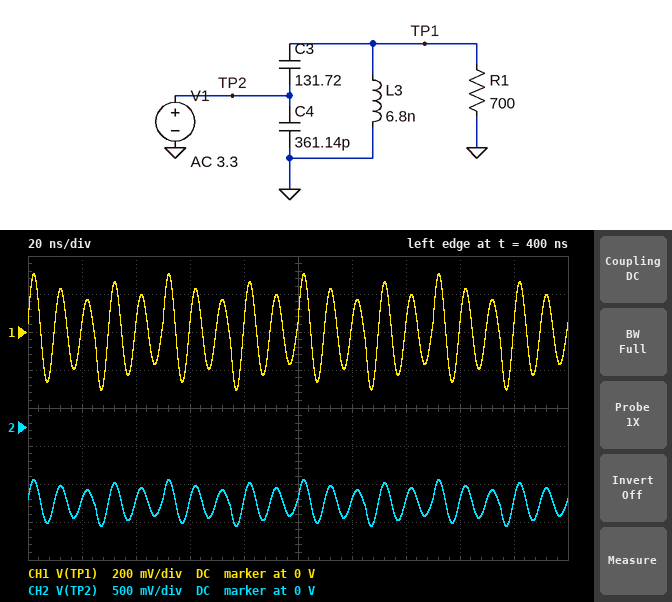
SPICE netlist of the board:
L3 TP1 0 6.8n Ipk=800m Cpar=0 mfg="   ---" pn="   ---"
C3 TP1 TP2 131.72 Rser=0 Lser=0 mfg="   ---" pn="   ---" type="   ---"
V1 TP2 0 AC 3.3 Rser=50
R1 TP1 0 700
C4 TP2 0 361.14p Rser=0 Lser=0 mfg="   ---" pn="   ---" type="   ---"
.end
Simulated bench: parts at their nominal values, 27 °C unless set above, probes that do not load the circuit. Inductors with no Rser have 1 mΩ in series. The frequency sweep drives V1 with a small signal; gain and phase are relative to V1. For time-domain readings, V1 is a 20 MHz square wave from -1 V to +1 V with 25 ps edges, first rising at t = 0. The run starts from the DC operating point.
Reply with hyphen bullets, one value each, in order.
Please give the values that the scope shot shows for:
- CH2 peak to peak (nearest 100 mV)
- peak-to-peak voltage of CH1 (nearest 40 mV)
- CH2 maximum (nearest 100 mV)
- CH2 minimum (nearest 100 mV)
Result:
- 600 mV
- 600 mV
- -700 mV
- -1.3 V
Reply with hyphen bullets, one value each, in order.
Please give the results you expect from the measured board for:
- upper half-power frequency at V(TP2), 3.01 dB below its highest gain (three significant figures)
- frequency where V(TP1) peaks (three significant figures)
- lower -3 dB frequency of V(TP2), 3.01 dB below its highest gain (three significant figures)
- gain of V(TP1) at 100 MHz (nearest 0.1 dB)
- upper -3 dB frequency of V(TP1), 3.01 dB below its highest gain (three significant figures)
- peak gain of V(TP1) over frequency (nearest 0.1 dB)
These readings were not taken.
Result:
- 106 MHz
- 102 MHz
- 96.9 MHz
- -1.1 dB
- 106 MHz
- -0.6 dB
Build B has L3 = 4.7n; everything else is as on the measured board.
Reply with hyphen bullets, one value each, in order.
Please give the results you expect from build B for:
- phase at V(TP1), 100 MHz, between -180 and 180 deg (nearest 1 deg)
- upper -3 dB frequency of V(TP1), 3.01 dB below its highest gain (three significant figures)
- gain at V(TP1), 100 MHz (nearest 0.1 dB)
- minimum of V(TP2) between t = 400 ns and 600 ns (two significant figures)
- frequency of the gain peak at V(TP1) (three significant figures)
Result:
- 79 deg
- 127 MHz
- -15.1 dB
- -1.1 V
- 122 MHz
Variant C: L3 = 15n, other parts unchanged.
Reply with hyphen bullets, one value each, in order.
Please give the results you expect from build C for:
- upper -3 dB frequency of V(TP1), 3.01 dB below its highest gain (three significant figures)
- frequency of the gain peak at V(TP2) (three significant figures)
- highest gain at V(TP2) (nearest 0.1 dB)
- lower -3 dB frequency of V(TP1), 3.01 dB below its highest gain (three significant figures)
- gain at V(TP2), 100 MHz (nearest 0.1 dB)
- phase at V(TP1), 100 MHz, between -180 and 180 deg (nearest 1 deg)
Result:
- 73.3 MHz
- 68.4 MHz
- -0.6 dB
- 63.8 MHz
- -15.8 dB
- -80 deg
